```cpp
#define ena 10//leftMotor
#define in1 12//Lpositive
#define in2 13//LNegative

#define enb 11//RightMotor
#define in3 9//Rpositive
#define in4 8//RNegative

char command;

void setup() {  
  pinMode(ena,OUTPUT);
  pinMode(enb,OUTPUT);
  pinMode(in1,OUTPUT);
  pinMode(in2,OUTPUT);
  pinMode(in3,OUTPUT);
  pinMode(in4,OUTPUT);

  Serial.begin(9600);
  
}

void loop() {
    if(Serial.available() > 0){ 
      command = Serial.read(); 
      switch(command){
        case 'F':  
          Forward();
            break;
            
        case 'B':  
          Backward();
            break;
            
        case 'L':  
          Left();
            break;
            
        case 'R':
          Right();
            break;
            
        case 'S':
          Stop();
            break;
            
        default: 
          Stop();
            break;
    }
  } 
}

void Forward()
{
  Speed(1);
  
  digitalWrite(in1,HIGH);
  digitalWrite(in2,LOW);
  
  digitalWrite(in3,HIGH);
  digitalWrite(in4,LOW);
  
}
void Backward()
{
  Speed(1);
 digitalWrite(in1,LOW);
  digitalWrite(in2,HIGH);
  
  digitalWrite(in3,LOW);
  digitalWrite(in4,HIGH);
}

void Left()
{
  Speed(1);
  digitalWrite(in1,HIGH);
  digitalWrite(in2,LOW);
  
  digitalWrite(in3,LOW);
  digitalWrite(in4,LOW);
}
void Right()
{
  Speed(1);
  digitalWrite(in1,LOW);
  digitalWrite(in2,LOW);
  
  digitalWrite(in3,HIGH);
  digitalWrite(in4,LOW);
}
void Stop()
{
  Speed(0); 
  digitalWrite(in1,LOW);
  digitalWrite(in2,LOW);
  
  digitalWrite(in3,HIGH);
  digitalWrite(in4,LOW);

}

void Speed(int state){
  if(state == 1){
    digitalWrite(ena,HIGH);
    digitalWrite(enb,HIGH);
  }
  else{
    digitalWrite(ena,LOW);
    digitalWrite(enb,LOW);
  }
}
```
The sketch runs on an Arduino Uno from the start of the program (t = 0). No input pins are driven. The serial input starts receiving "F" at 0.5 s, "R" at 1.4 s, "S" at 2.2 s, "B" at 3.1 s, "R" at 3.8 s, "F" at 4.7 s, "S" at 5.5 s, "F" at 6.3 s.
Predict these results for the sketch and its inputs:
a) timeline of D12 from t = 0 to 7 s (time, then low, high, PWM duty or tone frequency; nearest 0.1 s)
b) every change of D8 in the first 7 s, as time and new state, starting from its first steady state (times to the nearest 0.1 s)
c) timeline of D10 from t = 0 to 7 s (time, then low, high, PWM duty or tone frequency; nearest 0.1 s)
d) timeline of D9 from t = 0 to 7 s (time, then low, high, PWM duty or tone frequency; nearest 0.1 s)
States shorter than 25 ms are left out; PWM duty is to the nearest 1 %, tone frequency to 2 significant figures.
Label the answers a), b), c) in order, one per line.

a) 0 s low; 0.5 s high; 1.4 s low; 4.7 s high; 5.5 s low; 6.3 s high
b) 0 s low; 3.1 s high; 3.8 s low
c) 0 s low; 0.5 s high; 2.2 s low; 3.1 s high; 5.5 s low; 6.3 s high
d) 0 s low; 0.5 s high; 3.1 s low; 3.8 s high
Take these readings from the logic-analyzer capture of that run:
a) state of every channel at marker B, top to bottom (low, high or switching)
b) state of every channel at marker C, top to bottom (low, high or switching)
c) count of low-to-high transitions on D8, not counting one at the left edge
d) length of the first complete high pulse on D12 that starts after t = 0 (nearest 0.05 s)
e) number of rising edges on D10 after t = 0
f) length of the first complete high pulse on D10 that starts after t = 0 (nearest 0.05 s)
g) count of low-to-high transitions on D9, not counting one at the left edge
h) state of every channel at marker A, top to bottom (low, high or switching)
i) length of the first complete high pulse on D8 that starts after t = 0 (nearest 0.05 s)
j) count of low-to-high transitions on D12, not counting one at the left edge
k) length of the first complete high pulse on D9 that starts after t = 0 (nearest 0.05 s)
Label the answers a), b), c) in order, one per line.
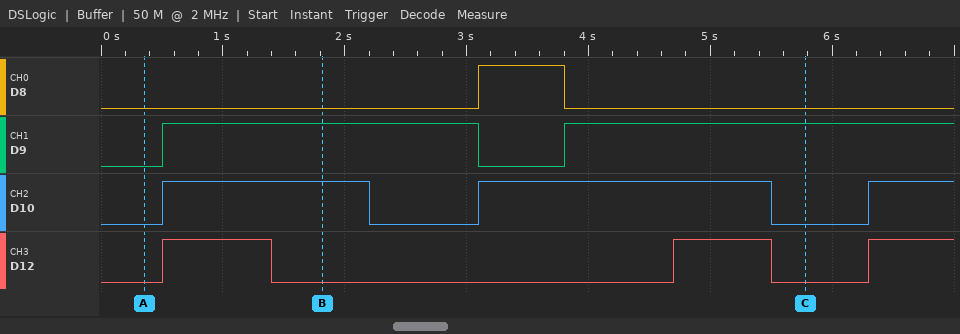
a) D8 low, D9 high, D10 high, D12 low
b) D8 low, D9 high, D10 low, D12 low
c) 1
d) 0.90 s
e) 3
f) 1.70 s
g) 2
h) D8 low, D9 low, D10 low, D12 low
i) 0.70 s
j) 3
k) 2.60 s
